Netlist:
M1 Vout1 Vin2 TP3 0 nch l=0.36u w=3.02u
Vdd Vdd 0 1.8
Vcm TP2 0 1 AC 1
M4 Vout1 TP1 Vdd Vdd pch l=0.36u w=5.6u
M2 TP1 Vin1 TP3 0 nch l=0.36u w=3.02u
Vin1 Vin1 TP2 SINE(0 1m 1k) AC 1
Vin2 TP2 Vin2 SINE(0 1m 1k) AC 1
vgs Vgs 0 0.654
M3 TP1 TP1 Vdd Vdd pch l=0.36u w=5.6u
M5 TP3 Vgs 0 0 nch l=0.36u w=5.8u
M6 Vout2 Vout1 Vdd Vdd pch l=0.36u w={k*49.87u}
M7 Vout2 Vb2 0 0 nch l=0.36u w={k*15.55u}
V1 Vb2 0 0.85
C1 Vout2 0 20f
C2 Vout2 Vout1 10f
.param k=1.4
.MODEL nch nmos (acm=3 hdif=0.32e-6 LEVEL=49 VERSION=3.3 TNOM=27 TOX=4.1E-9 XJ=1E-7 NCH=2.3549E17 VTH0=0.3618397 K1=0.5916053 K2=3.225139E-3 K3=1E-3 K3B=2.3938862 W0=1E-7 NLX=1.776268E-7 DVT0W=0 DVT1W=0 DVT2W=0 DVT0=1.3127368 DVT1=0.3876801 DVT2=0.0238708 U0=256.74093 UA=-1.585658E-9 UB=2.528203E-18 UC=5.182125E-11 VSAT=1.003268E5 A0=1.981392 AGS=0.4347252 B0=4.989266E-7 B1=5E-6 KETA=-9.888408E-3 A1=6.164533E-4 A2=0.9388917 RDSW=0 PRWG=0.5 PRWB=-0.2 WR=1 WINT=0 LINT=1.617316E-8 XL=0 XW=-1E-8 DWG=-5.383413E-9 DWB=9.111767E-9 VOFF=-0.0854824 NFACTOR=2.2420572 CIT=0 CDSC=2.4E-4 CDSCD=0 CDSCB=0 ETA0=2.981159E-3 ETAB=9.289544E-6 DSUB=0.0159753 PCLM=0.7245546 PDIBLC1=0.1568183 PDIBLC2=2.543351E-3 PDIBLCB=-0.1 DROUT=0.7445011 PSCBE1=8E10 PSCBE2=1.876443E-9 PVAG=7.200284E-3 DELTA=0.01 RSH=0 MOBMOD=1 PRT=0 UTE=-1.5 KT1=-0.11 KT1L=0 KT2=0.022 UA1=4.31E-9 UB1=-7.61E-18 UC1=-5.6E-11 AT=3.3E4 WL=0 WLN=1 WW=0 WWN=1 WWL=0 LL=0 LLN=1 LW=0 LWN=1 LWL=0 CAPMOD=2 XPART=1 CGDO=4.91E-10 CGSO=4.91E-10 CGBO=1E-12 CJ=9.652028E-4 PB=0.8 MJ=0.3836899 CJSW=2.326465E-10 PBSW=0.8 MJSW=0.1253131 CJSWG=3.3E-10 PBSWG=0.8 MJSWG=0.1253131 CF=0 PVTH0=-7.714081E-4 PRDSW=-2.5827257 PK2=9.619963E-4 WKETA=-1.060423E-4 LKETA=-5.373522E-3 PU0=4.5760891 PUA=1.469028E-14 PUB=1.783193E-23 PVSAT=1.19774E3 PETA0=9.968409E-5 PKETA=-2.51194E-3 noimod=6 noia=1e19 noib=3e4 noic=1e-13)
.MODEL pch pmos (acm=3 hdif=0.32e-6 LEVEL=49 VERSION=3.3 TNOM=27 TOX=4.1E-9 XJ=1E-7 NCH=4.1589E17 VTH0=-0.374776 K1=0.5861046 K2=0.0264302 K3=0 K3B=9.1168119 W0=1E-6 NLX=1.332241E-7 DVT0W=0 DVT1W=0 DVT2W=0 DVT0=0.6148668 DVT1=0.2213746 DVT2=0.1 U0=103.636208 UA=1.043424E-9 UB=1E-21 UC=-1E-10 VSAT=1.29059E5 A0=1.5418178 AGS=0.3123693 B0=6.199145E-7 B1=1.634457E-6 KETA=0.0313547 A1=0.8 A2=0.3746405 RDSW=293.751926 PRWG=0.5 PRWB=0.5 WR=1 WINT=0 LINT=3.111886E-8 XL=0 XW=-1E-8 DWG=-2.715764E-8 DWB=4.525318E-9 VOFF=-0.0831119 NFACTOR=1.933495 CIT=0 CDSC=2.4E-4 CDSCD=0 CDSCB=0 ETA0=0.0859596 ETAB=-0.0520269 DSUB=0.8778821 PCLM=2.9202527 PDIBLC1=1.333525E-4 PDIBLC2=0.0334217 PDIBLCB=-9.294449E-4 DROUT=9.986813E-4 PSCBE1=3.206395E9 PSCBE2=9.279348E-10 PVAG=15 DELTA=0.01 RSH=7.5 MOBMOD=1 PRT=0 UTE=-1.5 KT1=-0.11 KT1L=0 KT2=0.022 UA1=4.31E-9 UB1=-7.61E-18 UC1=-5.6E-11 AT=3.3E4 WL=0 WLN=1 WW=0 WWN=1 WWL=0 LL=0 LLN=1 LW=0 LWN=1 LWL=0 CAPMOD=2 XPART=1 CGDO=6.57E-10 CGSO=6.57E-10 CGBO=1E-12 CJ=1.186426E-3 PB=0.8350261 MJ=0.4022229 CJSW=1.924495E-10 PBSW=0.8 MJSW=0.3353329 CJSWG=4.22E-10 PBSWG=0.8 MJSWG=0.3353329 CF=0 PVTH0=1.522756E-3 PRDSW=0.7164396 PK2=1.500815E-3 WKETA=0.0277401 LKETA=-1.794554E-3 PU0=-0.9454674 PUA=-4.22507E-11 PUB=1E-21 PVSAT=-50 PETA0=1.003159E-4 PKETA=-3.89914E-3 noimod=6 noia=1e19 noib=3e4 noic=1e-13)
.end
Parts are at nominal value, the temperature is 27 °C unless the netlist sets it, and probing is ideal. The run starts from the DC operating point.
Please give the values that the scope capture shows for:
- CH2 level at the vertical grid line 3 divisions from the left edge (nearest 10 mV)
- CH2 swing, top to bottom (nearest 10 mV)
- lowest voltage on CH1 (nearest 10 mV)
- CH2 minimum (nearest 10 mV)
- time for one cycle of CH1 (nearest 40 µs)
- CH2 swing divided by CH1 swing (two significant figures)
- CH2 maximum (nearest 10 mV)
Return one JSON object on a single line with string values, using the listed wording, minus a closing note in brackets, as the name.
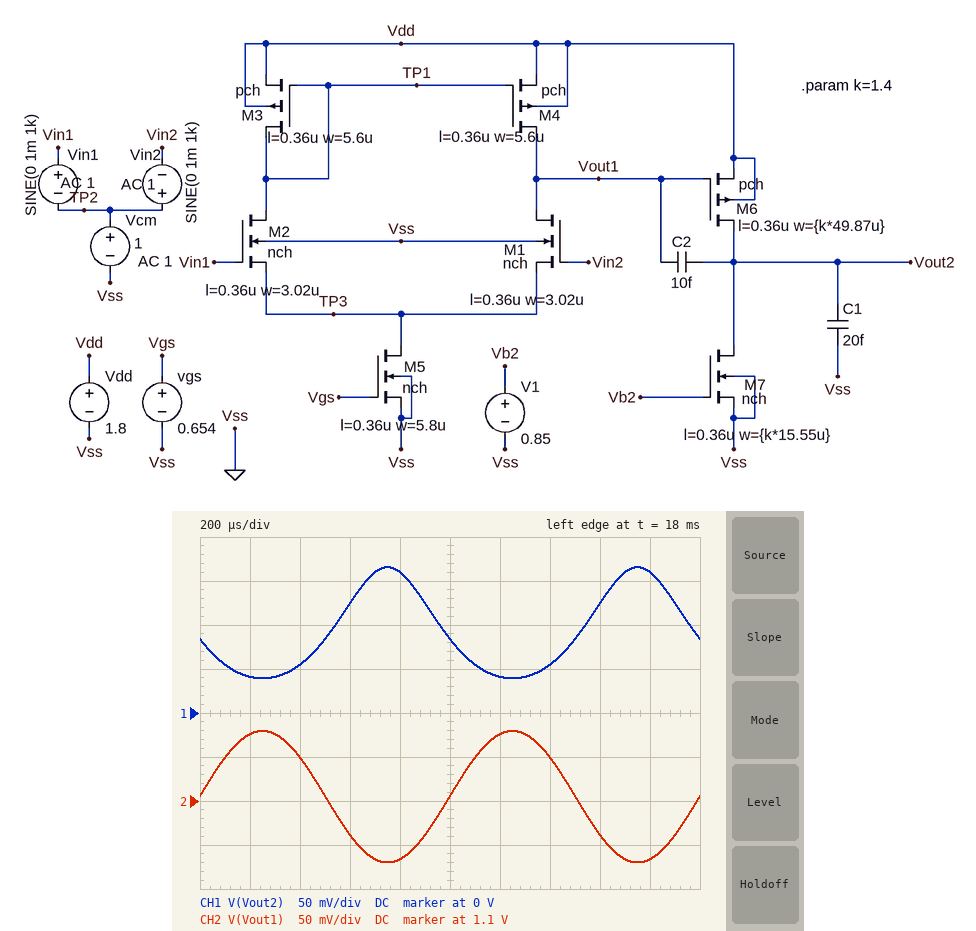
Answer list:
{"CH2 level at the vertical grid line 3 divisions from the left edge": "1.06 V", "CH2 swing, top to bottom": "150 mV", "lowest voltage on CH1": "40 mV", "CH2 minimum": "1.03 V", "time for one cycle of CH1": "1.00 ms", "CH2 swing divided by CH1 swing": "1.2", "CH2 maximum": "1.18 V"}
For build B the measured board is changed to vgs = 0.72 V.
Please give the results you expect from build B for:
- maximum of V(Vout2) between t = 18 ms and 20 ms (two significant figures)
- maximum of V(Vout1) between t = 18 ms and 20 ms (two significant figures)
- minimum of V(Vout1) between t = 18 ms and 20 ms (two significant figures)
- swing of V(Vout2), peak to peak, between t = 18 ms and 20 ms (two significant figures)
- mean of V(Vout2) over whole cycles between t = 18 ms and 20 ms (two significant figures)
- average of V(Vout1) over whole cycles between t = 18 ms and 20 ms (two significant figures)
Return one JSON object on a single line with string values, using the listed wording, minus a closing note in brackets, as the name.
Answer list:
{"maximum of V(Vout2) between t = 18 ms and 20 ms": "920 mV", "maximum of V(Vout1) between t = 18 ms and 20 ms": "1.1 V", "minimum of V(Vout1) between t = 18 ms and 20 ms": "950 mV", "swing of V(Vout2), peak to peak, between t = 18 ms and 20 ms": "820 mV", "mean of V(Vout2) over whole cycles between t = 18 ms and 20 ms": "320 mV", "average of V(Vout1) over whole cycles between t = 18 ms and 20 ms": "1.0 V"}
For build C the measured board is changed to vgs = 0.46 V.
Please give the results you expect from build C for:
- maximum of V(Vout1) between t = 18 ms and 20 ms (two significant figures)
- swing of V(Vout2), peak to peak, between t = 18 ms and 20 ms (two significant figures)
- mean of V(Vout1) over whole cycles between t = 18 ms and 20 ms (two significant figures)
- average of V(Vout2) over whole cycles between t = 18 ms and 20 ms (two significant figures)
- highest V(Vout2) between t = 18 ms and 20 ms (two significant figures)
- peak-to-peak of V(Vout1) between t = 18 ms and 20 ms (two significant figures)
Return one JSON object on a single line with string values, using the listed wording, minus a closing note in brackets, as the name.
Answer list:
{"maximum of V(Vout1) between t = 18 ms and 20 ms": "1.4 V", "swing of V(Vout2), peak to peak, between t = 18 ms and 20 ms": "13 mV", "mean of V(Vout1) over whole cycles between t = 18 ms and 20 ms": "1.3 V", "average of V(Vout2) over whole cycles between t = 18 ms and 20 ms": "5.2 mV", "highest V(Vout2) between t = 18 ms and 20 ms": "14 mV", "peak-to-peak of V(Vout1) between t = 18 ms and 20 ms": "160 mV"}
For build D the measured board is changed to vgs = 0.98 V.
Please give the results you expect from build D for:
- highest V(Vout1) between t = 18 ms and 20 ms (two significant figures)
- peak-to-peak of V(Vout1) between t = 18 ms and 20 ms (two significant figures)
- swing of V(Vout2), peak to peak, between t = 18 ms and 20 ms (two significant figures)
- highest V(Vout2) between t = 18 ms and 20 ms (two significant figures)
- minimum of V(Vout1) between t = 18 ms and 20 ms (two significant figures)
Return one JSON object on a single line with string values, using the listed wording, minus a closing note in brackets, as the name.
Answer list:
{"highest V(Vout1) between t = 18 ms and 20 ms": "890 mV", "peak-to-peak of V(Vout1) between t = 18 ms and 20 ms": "110 mV", "swing of V(Vout2), peak to peak, between t = 18 ms and 20 ms": "82 mV", "highest V(Vout2) between t = 18 ms and 20 ms": "1.6 V", "minimum of V(Vout1) between t = 18 ms and 20 ms": "780 mV"}
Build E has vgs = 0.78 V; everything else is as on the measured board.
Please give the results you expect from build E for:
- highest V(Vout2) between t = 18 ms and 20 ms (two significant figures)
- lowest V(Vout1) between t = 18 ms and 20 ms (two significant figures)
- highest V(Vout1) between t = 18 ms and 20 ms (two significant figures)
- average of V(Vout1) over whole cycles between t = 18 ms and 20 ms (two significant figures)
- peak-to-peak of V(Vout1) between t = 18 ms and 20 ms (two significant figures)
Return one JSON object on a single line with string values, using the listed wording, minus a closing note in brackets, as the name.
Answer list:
{"highest V(Vout2) between t = 18 ms and 20 ms": "1.5 V", "lowest V(Vout1) between t = 18 ms and 20 ms": "890 mV", "highest V(Vout1) between t = 18 ms and 20 ms": "1.0 V", "average of V(Vout1) over whole cycles between t = 18 ms and 20 ms": "950 mV", "peak-to-peak of V(Vout1) between t = 18 ms and 20 ms": "120 mV"}
